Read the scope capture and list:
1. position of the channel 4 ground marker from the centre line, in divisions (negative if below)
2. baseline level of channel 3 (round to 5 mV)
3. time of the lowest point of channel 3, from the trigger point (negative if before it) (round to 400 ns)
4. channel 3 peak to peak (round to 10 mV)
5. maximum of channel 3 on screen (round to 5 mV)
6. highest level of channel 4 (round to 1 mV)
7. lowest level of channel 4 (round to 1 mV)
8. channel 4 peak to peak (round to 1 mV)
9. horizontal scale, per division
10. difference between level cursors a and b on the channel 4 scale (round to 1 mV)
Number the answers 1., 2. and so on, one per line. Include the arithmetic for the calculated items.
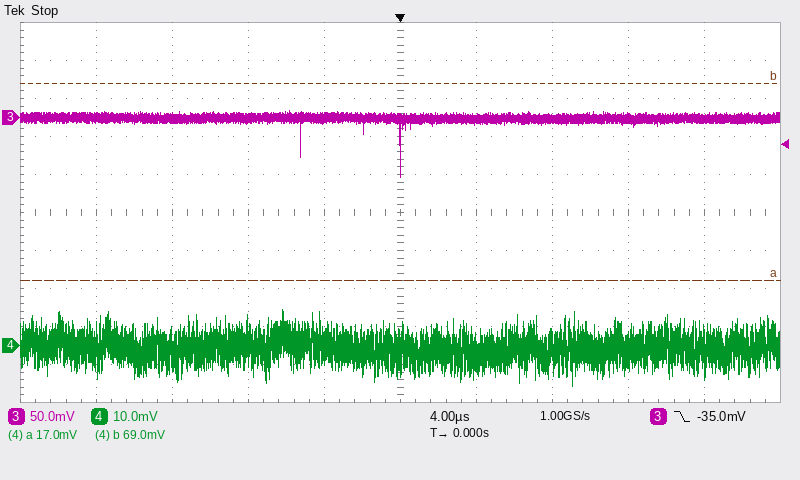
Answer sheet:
1. -3.5 div
2. 0 mV
3. 0.0 µs
4. 90 mV
5. 10 mV
6. 9 mV
7. -11 mV
8. 9 mV − (-11 mV) = 20 mV
9. 4 µs
10. 52 mV
